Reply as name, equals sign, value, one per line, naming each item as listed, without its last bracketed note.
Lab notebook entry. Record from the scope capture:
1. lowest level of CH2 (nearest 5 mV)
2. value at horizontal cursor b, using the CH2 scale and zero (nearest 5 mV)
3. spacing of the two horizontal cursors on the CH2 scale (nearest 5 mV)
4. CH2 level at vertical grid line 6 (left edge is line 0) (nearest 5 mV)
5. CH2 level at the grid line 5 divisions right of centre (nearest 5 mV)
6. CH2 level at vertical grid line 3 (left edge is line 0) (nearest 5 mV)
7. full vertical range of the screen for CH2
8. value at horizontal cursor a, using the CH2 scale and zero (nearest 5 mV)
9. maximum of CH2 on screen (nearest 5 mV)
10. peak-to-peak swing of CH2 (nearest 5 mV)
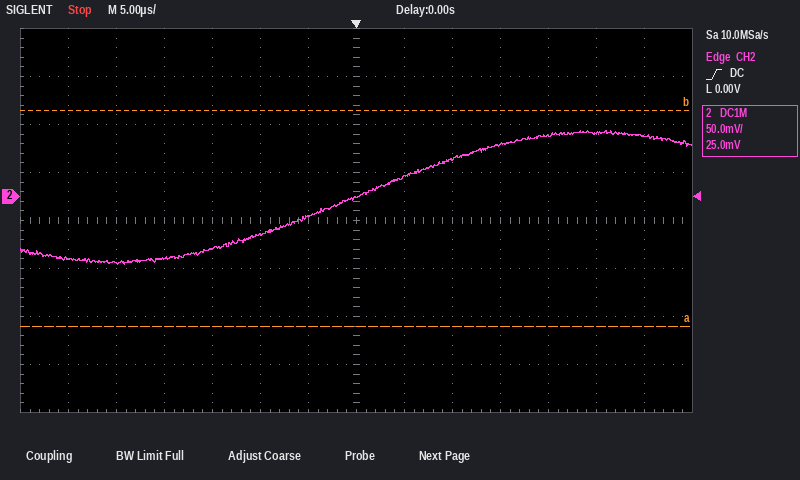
lowest level of CH2 = -70 mV
value at horizontal cursor b, using the CH2 scale and zero = 90 mV
spacing of the two horizontal cursors on the CH2 scale = 225 mV
CH2 level at vertical grid line 6 (left edge is line 0) = -20 mV
CH2 level at the grid line 5 divisions right of centre = 65 mV
CH2 level at vertical grid line 3 (left edge is line 0) = -65 mV
full vertical range of the screen for CH2 = 400 mV
value at horizontal cursor a, using the CH2 scale and zero = -135 mV
maximum of CH2 on screen = 70 mV
peak-to-peak swing of CH2 = 140 mV
